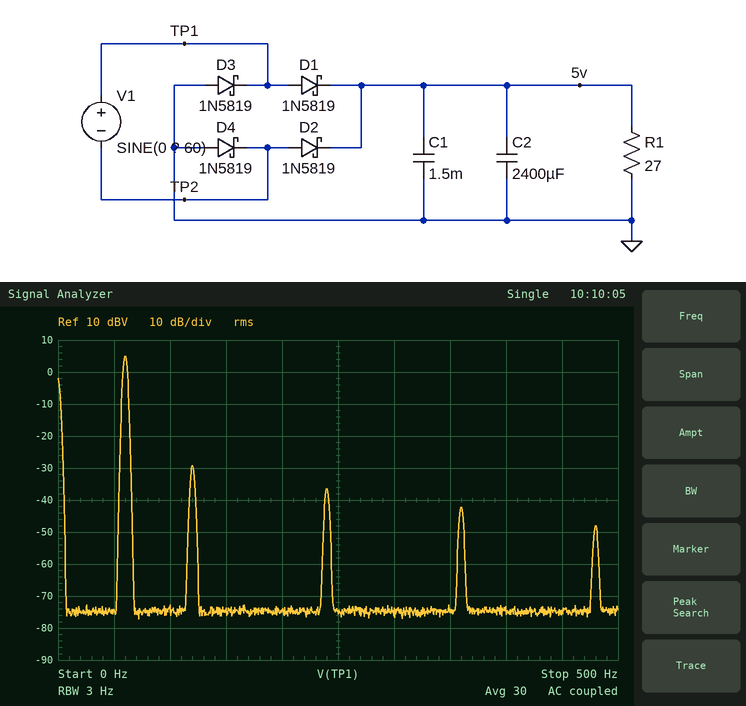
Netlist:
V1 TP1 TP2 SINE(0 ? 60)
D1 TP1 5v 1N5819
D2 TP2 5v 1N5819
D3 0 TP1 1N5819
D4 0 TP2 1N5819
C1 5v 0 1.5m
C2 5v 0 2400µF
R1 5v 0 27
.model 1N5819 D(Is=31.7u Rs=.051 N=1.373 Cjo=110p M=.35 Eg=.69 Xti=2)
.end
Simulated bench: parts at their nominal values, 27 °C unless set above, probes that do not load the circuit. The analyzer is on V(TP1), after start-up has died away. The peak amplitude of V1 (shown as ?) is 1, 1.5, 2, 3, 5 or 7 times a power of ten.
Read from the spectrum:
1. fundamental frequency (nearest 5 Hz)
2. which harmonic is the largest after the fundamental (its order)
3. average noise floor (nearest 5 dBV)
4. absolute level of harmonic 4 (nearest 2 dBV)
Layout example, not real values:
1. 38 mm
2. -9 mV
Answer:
1. 60 Hz
2. 2
3. -75 dBV
4. -36 dBV
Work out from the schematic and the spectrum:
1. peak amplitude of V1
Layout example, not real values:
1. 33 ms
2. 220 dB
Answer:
1. 5 V
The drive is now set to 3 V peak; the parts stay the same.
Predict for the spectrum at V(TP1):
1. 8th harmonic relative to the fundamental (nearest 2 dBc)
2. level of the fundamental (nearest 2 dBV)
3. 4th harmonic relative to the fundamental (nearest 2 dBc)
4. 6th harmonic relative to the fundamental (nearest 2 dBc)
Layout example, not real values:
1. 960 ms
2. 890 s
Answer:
1. -56 dBc
2. 0 dBV
3. -42 dBc
4. -50 dBc
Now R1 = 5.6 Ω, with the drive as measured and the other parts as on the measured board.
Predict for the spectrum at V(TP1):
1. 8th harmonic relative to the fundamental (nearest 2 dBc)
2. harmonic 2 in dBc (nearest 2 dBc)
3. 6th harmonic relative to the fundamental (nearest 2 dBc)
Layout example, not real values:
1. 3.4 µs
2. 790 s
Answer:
1. -50 dBc
2. -22 dBc
3. -40 dBc
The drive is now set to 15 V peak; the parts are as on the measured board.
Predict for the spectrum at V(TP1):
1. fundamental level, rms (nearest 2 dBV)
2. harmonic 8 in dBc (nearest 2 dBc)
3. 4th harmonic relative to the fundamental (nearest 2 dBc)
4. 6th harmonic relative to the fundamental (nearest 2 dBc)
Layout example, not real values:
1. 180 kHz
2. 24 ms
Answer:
1. 14 dBV
2. -50 dBc
3. -40 dBc
4. -46 dBc
